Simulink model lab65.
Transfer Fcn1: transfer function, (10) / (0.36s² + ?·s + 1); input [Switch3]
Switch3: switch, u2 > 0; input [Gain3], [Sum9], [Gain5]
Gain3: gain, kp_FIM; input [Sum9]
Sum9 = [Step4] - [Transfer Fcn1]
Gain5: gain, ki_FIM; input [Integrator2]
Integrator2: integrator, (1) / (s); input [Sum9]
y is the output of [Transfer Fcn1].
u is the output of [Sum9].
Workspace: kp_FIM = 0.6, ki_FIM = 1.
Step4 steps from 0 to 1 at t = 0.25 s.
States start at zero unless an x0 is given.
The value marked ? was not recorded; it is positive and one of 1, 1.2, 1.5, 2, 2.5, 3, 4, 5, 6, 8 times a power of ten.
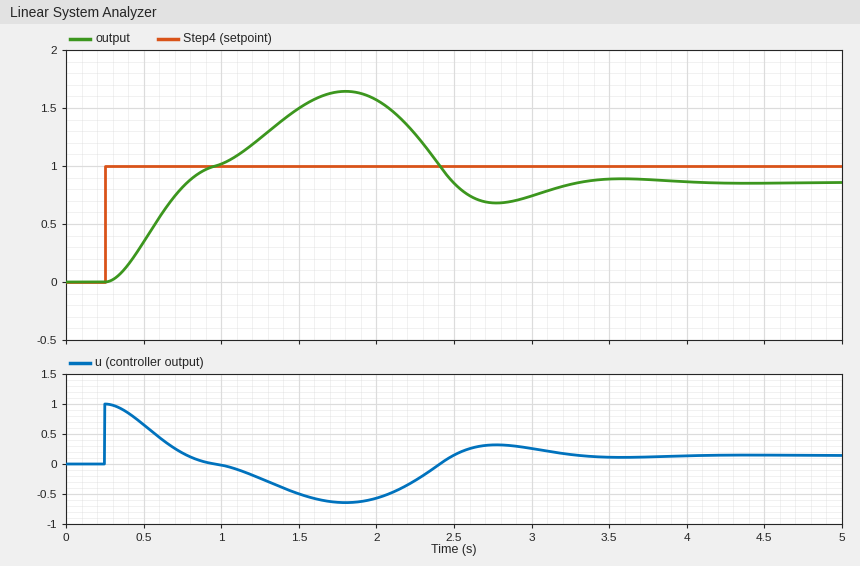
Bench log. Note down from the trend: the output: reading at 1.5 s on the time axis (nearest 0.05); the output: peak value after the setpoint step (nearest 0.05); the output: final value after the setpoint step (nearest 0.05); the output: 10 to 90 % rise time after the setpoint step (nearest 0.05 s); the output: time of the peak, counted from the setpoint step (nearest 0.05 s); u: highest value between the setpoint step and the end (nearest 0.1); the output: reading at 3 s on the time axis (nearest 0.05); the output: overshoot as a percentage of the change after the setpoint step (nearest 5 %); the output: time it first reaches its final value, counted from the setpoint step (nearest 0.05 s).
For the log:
1.50
1.65
0.85
0.35 s
1.55 s
1.0
0.75
90 %
0.55 s
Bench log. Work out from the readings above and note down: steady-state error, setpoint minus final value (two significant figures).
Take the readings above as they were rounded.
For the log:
0.15
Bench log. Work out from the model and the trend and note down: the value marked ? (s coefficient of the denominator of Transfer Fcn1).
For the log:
1.5
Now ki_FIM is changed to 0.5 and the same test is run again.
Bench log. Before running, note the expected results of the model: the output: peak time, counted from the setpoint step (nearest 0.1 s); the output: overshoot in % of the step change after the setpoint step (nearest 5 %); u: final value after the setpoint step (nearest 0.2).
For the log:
1.6 s
45 %
0.2
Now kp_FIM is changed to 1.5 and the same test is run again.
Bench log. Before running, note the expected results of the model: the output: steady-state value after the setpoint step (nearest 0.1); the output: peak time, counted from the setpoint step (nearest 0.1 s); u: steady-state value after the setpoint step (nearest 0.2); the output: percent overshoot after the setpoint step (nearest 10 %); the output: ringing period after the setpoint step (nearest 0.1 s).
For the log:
0.9
0.8 s
0.0
70 %
1.3 s
